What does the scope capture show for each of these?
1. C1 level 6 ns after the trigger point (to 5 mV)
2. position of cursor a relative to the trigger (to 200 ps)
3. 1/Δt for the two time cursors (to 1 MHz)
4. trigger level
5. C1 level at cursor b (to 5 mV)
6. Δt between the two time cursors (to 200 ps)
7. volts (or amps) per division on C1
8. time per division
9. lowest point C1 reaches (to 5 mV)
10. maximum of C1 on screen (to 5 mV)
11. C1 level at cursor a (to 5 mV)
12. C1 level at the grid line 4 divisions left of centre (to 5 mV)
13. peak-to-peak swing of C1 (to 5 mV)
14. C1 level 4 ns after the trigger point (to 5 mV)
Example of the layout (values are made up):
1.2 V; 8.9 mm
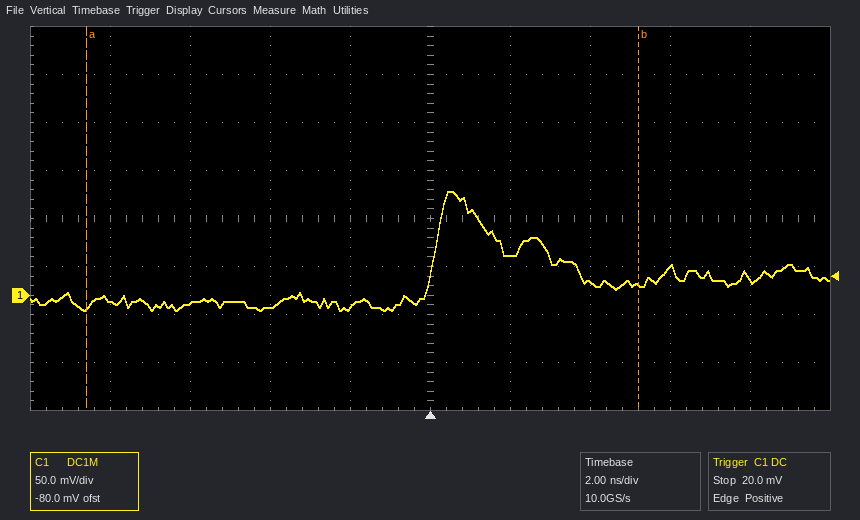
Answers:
30 mV; -8.6 ns; 72 MHz; 20.0 mV; 10 mV; 13.8 ns; 50 mV; 2 ns; -15 mV; 110 mV; -15 mV; -5 mV; 125 mV; 15 mV
